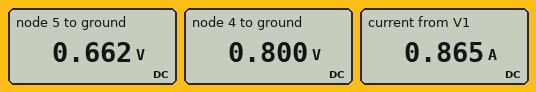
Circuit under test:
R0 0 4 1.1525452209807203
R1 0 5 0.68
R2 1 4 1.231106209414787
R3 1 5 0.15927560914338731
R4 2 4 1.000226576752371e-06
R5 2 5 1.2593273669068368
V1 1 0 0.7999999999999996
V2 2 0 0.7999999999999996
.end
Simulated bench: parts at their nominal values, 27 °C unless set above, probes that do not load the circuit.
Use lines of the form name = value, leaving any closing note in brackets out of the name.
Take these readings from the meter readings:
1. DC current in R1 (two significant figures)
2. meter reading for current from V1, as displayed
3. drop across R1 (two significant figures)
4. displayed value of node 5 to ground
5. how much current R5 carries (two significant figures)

DC current in R1 = 970 mA
meter reading for current from V1, as displayed = 0.865 A
drop across R1 = 660 mV
displayed value of node 5 to ground = 0.662 V
how much current R5 carries = 110 mA
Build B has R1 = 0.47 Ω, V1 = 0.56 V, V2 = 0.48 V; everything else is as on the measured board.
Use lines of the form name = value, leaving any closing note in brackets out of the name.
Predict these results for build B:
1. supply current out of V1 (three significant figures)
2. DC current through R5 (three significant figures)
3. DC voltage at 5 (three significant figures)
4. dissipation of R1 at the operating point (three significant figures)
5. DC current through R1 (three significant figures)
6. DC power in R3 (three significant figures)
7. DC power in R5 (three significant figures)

supply current out of V1 = 921 mA
DC current through R5 = 44.8 mA
DC voltage at 5 = 424 mV
dissipation of R1 at the operating point = 382 mW
DC current through R1 = 901 mA
DC power in R3 = 117 mW
DC power in R5 = 2.53 mW
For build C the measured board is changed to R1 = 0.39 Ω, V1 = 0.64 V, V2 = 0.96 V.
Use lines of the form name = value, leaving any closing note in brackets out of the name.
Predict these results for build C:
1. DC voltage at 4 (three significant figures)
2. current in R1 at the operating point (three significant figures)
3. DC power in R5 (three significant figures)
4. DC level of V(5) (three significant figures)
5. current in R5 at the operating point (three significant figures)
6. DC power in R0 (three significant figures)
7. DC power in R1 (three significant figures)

DC voltage at 4 = 960 mV
current in R1 at the operating point = 1.27 A
DC power in R5 = 171 mW
DC level of V(5) = 496 mV
current in R5 at the operating point = 368 mA
DC power in R0 = 800 mW
DC power in R1 = 631 mW
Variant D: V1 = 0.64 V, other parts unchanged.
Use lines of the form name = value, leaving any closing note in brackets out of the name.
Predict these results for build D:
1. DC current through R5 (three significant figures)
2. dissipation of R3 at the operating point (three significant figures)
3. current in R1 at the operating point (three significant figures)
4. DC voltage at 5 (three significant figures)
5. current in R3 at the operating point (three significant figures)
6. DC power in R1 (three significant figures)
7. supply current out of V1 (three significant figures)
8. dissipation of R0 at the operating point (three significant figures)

DC current through R5 = 203 mA
dissipation of R3 at the operating point = 57.0 mW
current in R1 at the operating point = 801 mA
DC voltage at 5 = 545 mV
current in R3 at the operating point = 598 mA
DC power in R1 = 436 mW
supply current out of V1 = 468 mA
dissipation of R0 at the operating point = 555 mW
